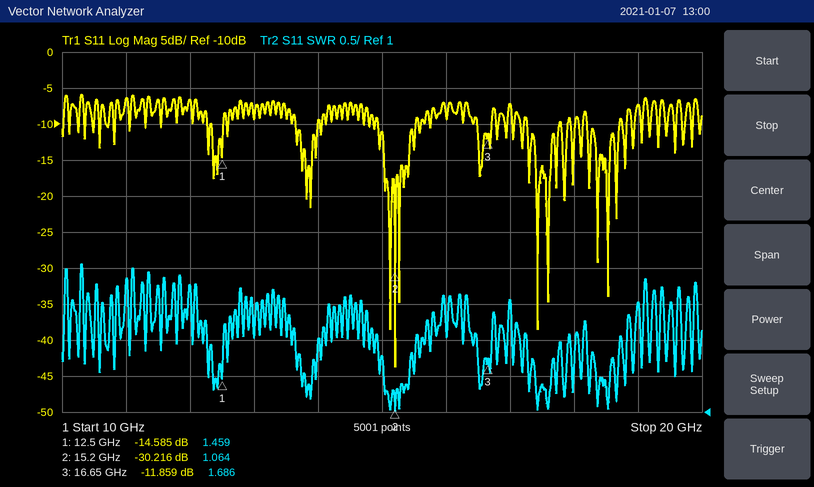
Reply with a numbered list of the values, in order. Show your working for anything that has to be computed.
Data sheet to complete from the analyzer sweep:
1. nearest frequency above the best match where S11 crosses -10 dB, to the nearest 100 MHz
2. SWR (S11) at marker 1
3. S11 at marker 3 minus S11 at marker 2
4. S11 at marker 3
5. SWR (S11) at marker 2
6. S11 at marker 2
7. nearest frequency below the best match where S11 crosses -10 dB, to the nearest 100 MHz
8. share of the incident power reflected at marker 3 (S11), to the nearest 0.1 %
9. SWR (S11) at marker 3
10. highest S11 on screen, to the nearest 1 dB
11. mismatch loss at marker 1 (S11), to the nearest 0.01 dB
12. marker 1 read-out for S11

1. 15.5 GHz
2. 1.459
3. -11.859 − (-30.216) = 18.357 dB
4. -11.859 dB
5. 1.064
6. -30.216 dB
7. 14.9 GHz
8. 10^(-11.859/10) ≈ 6.5 %
9. 1.686
10. -6 dB
11. −10 log10(1 − 10^(-14.585/10)) ≈ 0.15 dB
12. -14.585 dB
